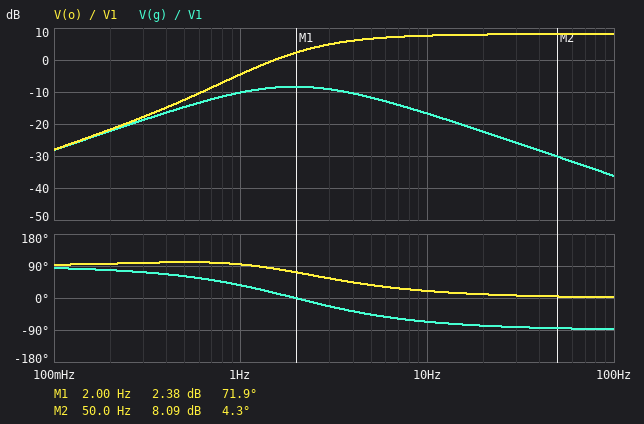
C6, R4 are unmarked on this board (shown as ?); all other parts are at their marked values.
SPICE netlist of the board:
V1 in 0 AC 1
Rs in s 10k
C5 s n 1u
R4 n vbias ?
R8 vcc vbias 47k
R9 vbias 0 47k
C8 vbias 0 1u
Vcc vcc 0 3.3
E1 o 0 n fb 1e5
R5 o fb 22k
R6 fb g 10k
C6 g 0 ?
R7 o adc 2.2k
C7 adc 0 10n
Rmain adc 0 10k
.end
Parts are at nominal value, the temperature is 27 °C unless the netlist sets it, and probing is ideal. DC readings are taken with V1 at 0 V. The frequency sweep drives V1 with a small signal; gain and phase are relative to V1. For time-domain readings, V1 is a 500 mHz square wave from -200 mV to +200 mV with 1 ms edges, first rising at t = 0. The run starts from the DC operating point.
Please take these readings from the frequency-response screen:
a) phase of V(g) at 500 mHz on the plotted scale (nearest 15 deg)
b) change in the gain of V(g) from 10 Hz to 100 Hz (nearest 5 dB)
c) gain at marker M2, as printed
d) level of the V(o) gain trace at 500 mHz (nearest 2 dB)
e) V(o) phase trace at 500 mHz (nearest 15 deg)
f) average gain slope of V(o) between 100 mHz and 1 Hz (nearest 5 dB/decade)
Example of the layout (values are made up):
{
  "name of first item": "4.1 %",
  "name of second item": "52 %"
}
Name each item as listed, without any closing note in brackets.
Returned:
{
  "phase of V(g) at 500 mHz on the plotted scale": "60 deg",
  "change in the gain of V(g) from 10 Hz to 100 Hz": "-20 dB",
  "gain at marker M2, as printed": "8.09 dB",
  "level of the V(o) gain trace at 500 mHz": "-12 dB",
  "V(o) phase trace at 500 mHz": "105 deg",
  "average gain slope of V(o) between 100 mHz and 1 Hz": "25 dB/decade"
}
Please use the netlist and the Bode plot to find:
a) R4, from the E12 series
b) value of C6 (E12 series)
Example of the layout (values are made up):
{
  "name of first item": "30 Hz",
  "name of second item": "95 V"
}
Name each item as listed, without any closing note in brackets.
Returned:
{
  "R4, from the E12 series": "39 kΩ",
  "value of C6": "8.2 µF"
}
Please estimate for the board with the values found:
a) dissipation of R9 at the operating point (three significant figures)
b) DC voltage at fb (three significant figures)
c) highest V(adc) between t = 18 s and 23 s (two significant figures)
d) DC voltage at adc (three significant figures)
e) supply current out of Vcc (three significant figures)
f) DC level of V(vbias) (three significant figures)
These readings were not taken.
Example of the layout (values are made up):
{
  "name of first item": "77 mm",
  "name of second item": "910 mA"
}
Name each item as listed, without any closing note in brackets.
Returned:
{
  "dissipation of R9 at the operating point": "57.9 µW",
  "DC voltage at fb": "1.65 V",
  "highest V(adc) between t = 18 s and 23 s": "2.2 V",
  "DC voltage at adc": "1.35 V",
  "supply current out of Vcc": "35.1 µA",
  "DC level of V(vbias)": "1.65 V"
}
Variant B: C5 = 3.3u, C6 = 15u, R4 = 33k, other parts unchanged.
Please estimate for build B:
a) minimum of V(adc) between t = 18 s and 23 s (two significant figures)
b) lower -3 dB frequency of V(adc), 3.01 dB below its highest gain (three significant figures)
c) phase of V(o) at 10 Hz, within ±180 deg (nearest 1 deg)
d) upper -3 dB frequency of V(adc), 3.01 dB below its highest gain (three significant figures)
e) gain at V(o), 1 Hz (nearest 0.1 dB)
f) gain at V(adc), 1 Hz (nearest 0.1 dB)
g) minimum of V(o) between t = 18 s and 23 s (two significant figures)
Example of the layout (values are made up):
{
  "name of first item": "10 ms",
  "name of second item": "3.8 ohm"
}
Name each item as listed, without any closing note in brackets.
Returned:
{
  "minimum of V(adc) between t = 18 s and 23 s": "540 mV",
  "lower -3 dB frequency of V(adc), 3.01 dB below its highest gain": "1.24 Hz",
  "phase of V(o) at 10 Hz, within ±180 deg": "6 deg",
  "upper -3 dB frequency of V(adc), 3.01 dB below its highest gain": "8.30 kHz",
  "gain at V(o), 1 Hz": "3.8 dB",
  "gain at V(adc), 1 Hz": "2.1 dB",
  "minimum of V(o) between t = 18 s and 23 s": "660 mV"
}
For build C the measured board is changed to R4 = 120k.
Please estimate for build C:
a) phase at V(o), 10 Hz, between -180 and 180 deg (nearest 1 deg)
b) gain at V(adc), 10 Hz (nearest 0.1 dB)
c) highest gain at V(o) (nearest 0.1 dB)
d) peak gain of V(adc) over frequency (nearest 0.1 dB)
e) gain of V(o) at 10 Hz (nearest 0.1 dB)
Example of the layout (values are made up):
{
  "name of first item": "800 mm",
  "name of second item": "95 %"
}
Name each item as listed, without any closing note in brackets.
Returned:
{
  "phase at V(o), 10 Hz, between -180 and 180 deg": "14 deg",
  "gain at V(adc), 10 Hz": "7.4 dB",
  "highest gain at V(o)": "9.4 dB",
  "peak gain of V(adc) over frequency": "7.7 dB",
  "gain of V(o) at 10 Hz": "9.2 dB"
}
